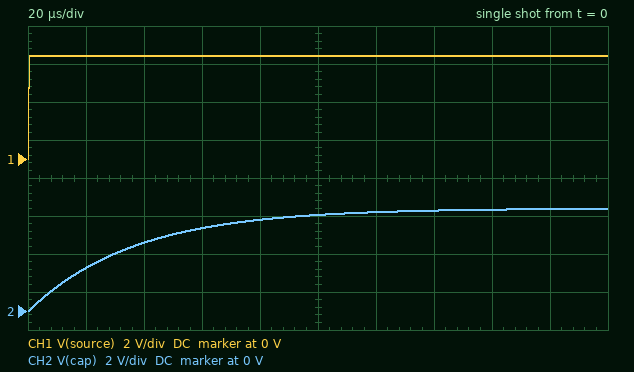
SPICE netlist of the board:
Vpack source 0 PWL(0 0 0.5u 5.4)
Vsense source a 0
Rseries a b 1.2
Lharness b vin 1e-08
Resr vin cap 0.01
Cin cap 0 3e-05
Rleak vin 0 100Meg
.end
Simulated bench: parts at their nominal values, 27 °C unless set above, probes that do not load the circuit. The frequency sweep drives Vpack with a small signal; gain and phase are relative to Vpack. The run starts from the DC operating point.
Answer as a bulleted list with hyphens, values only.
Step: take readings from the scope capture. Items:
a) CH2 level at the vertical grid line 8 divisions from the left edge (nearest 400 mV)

- 5.2 V
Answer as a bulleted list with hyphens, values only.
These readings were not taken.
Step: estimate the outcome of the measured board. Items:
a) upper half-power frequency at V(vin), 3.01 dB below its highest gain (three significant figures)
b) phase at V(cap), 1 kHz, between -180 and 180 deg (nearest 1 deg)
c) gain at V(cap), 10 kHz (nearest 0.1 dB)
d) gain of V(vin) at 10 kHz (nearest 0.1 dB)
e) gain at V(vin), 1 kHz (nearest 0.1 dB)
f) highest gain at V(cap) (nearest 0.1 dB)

- 4.39 kHz
- -13 deg
- -7.9 dB
- -7.9 dB
- -0.2 dB
- 0 dB
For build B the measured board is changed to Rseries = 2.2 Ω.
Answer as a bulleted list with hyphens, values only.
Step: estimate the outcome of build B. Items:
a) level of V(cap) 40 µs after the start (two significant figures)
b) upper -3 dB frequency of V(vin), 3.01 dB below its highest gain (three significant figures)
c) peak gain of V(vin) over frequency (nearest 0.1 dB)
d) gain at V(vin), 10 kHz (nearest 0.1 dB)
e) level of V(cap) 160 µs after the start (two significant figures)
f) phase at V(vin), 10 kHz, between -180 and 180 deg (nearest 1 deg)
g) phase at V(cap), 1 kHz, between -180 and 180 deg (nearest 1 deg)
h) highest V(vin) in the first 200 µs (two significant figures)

- 2.4 V
- 2.40 kHz
- 0 dB
- -12.6 dB
- 4.9 V
- -75 deg
- -23 deg
- 5.1 V
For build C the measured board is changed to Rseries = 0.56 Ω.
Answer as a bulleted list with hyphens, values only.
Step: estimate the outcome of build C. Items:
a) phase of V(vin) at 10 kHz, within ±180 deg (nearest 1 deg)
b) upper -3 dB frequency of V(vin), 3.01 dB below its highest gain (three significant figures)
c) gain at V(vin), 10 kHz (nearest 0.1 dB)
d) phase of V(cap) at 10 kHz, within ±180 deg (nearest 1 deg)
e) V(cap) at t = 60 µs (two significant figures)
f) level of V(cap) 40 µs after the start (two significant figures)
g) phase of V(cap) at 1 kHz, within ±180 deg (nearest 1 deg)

- -46 deg
- 9.32 kHz
- -3.3 dB
- -47 deg
- 5.2 V
- 4.9 V
- -6 deg
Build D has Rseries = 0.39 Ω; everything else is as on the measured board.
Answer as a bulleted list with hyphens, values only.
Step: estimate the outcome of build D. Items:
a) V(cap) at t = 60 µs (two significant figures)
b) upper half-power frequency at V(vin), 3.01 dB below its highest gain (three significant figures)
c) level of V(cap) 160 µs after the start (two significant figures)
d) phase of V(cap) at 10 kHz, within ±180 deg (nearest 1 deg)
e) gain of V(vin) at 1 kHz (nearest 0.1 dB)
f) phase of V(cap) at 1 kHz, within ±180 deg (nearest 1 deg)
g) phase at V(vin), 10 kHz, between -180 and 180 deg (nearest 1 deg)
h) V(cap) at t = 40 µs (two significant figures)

- 5.4 V
- 13.3 kHz
- 5.4 V
- -37 deg
- 0 dB
- -4 deg
- -36 deg
- 5.2 V
